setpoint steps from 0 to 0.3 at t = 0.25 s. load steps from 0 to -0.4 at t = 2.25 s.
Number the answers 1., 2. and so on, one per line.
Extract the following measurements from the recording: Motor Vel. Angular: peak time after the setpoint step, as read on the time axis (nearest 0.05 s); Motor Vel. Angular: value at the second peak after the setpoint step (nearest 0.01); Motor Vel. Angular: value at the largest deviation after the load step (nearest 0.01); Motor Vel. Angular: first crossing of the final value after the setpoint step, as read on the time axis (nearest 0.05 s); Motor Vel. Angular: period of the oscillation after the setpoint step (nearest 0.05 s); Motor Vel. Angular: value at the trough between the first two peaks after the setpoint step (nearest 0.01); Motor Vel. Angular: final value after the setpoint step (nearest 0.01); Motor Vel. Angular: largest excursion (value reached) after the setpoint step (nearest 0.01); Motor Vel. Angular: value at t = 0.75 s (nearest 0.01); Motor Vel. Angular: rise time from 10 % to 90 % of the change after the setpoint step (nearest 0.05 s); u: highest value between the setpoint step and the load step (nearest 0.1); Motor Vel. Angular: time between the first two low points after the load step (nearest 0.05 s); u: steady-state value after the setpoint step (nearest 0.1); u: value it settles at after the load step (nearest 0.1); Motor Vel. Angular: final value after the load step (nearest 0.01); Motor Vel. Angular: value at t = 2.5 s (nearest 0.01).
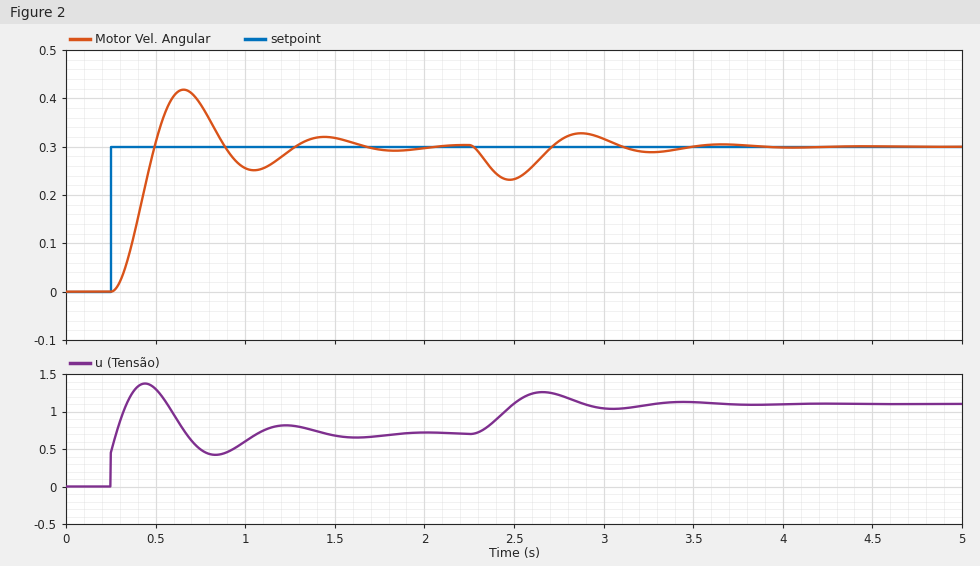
1. 0.65 s
2. 0.32
3. 0.23
4. 0.50 s
5. 0.80 s
6. 0.25
7. 0.30
8. 0.42
9. 0.39
10. 0.15 s
11. 1.4
12. 0.80 s
13. 0.7
14. 1.1
15. 0.30
16. 0.23
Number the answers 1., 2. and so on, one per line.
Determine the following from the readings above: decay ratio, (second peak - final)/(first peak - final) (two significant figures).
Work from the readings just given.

1. 0.17
